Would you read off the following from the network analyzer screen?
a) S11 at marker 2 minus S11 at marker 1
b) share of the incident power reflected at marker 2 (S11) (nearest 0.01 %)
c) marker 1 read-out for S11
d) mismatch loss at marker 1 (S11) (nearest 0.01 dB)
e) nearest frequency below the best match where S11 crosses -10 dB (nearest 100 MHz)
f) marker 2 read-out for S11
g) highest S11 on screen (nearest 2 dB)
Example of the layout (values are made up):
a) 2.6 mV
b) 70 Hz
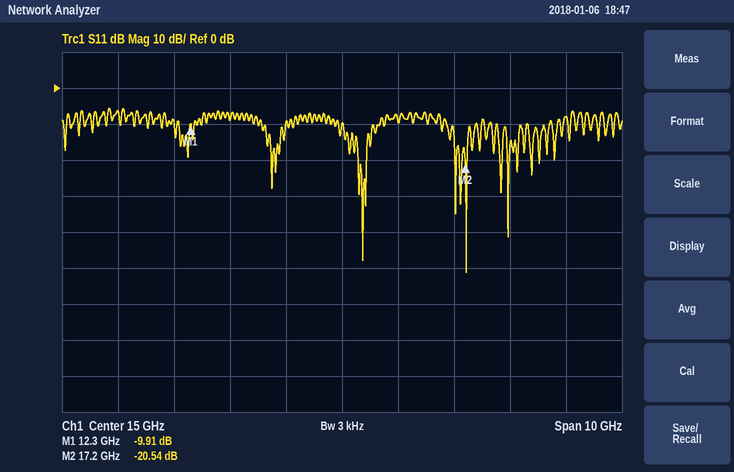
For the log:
a) -10.63 dB
b) 0.88 %
c) -9.91 dB
d) 0.47 dB
e) 16.9 GHz
f) -20.54 dB
g) -6 dB
